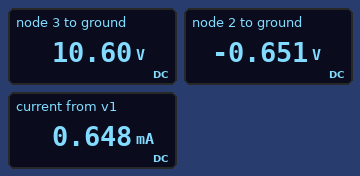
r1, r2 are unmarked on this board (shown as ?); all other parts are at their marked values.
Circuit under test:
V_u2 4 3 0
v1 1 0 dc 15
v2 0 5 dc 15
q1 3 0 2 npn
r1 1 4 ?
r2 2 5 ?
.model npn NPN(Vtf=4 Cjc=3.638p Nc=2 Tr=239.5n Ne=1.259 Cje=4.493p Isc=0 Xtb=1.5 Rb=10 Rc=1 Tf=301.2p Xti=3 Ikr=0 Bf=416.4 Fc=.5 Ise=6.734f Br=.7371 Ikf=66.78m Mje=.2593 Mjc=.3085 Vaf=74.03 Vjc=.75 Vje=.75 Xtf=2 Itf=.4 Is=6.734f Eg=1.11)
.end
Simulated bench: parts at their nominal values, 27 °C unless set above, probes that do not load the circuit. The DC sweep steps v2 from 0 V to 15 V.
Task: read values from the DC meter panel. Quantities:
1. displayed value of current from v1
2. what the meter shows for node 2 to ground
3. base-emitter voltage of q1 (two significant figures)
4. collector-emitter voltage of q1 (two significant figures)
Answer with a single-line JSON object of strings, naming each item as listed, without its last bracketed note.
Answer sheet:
{"displayed value of current from v1": "0.648 mA", "what the meter shows for node 2 to ground": "-0.651 V", "base-emitter voltage of q1": "650 mV", "collector-emitter voltage of q1": "11 V"}
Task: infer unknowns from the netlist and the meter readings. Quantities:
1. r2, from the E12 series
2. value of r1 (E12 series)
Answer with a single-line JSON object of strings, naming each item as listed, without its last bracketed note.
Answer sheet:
{"r2, from the E12 series": "22 kΩ", "value of r1": "6.8 kΩ"}
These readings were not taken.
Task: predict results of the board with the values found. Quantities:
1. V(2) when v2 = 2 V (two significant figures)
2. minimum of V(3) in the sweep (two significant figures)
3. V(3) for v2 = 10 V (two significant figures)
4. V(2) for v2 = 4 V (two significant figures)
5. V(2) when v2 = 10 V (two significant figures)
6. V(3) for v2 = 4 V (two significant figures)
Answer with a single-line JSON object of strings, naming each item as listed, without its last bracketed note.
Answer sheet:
{"V(2) when v2 = 2 V": "-590 mV", "minimum of V(3) in the sweep": "11 V", "V(3) for v2 = 10 V": "12 V", "V(2) for v2 = 4 V": "-610 mV", "V(2) when v2 = 10 V": "-640 mV", "V(3) for v2 = 4 V": "14 V"}
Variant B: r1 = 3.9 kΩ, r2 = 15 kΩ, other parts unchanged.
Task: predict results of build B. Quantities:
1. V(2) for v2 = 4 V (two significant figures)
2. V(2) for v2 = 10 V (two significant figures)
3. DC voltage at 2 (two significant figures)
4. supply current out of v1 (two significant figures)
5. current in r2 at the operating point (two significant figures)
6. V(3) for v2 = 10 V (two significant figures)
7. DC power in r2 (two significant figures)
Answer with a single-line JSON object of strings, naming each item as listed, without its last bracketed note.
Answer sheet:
{"V(2) for v2 = 4 V": "-620 mV", "V(2) for v2 = 10 V": "-650 mV", "DC voltage at 2": "-660 mV", "supply current out of v1": "950 µA", "current in r2 at the operating point": "960 µA", "V(3) for v2 = 10 V": "13 V", "DC power in r2": "14 mW"}
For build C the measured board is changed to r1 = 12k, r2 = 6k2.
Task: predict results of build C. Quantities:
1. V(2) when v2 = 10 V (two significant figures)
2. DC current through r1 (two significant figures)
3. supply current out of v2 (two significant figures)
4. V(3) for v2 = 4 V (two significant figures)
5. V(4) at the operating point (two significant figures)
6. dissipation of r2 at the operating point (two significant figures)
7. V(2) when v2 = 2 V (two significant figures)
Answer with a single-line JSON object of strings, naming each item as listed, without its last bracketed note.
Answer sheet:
{"V(2) when v2 = 10 V": "-680 mV", "DC current through r1": "1.3 mA", "supply current out of v2": "2.3 mA", "V(3) for v2 = 4 V": "8.6 V", "V(4) at the operating point": "-670 mV", "dissipation of r2 at the operating point": "33 mW", "V(2) when v2 = 2 V": "-620 mV"}
